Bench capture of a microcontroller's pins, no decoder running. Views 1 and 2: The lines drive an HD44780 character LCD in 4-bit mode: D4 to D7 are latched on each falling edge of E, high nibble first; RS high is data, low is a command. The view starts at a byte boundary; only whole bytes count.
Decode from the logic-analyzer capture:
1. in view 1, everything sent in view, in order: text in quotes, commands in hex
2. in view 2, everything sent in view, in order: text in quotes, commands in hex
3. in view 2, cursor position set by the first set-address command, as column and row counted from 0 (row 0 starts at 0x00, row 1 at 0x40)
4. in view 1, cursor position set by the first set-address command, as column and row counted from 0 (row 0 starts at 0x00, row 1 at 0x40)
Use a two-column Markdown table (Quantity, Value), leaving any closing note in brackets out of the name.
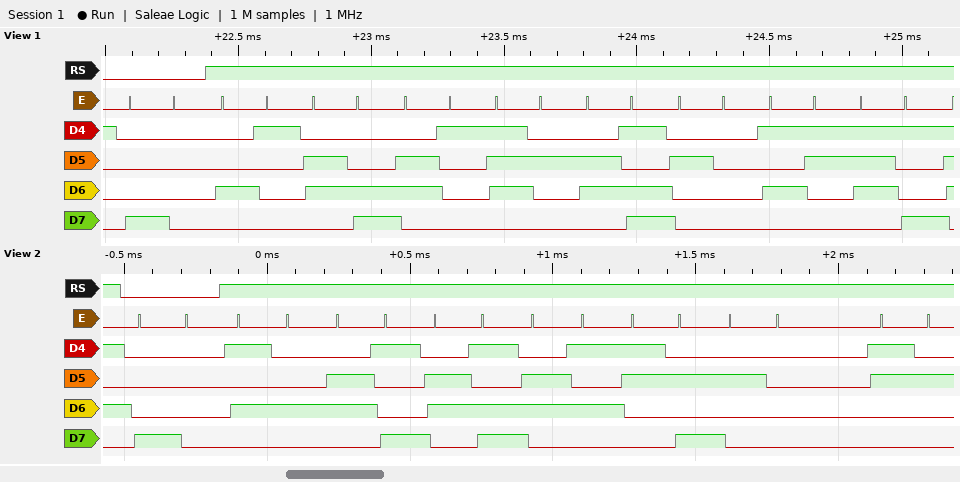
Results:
| Quantity | Value |
|---|---|
| in view 1, everything sent in view, in order: text in quotes, commands in hex | 0x80 "Alarm Sy" |
| in view 2, everything sent in view, in order: text in quotes, commands in hex | 0x80 "Time: 2" |
| in view 2, cursor position set by the first set-address command, as column and row counted from 0 | column 0, row 0 |
| in view 1, cursor position set by the first set-address command, as column and row counted from 0 | column 0, row 0 |
